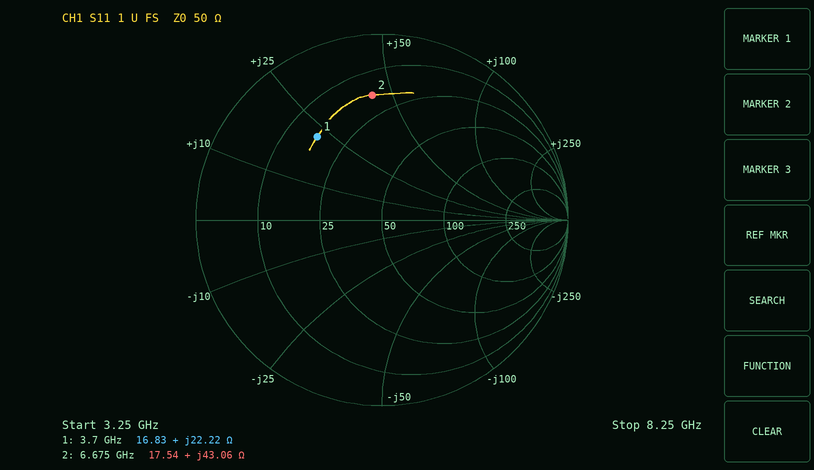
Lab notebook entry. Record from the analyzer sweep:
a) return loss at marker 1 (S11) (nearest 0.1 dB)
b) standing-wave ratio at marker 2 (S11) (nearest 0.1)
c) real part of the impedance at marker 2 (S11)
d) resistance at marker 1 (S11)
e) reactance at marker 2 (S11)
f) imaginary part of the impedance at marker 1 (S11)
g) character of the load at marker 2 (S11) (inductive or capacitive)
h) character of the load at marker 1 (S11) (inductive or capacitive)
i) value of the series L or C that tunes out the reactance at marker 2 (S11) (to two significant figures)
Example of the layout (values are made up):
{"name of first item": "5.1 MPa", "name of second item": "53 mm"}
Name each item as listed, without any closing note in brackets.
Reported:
{"return loss at marker 1 (S11)": "4.9 dB", "standing-wave ratio at marker 2 (S11)": "5.1", "real part of the impedance at marker 2": "17.54 Ω", "resistance at marker 1": "16.83 Ω", "reactance at marker 2": "+43.06 Ω", "imaginary part of the impedance at marker 1": "+22.22 Ω", "character of the load at marker 2 (S11)": "inductive", "character of the load at marker 1 (S11)": "inductive", "value of the series L or C that tunes out the reactance at marker 2 (S11)": "550 fF"}
